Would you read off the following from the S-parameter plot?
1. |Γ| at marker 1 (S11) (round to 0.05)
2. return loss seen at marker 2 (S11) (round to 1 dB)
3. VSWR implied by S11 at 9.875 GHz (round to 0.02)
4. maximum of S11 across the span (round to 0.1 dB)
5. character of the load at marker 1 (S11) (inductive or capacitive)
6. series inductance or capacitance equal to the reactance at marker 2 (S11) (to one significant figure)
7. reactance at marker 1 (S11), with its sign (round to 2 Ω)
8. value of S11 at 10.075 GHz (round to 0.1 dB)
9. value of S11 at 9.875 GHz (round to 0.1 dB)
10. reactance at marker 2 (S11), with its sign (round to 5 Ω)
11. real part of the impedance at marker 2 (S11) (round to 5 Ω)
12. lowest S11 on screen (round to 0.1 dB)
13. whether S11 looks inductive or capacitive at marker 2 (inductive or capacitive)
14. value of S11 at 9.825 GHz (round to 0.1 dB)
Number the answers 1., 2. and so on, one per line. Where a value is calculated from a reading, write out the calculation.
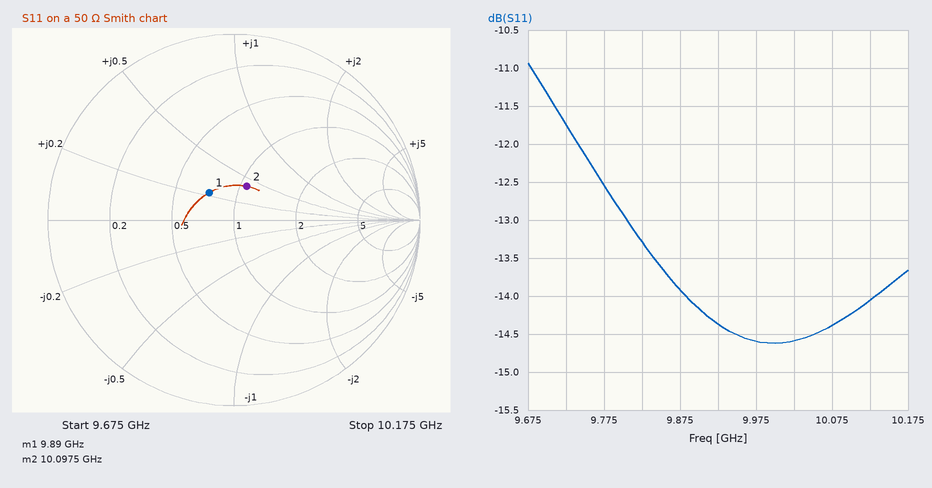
1. 0.20
2. 14 dB
3. |Γ| = 10^(-13.9/20) = 0.2018; VSWR = (1 + 0.2018)/(1 − 0.2018) ≈ 1.51, so 1.50 to the nearest 0.02
4. -10.9 dB
5. inductive
6. L = 20 Ω/(2π × 10.0975 GHz) ≈ 315 pH, so 300 pH to one significant figure
7. +12 Ω
8. -14.4 dB
9. -13.9 dB
10. +20 Ω
11. 55 Ω
12. -14.6 dB
13. inductive
14. -13.3 dB
